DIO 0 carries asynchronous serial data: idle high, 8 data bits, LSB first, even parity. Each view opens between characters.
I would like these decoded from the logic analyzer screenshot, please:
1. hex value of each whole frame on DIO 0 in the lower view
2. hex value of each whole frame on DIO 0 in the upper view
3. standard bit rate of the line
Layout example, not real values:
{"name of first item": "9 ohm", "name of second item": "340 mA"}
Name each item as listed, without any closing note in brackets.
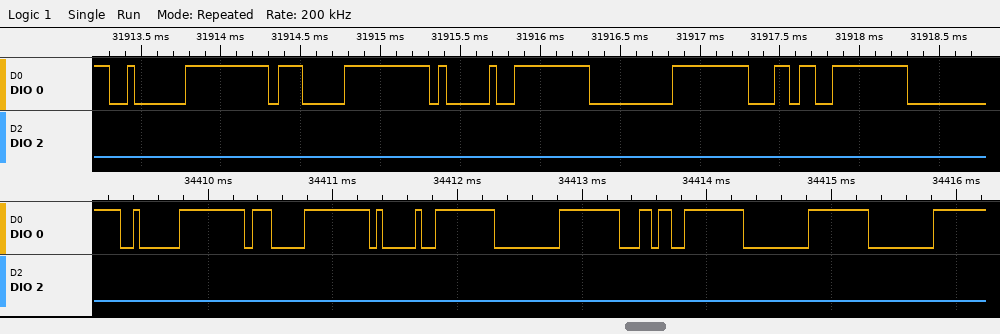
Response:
{"hex value of each whole frame on DIO 0 in the lower view": "02, 07, 41, 00, 6C, 00, 00", "hex value of each whole frame on DIO 0 in the upper view": "02, 07, 41, 00, 6C", "standard bit rate of the line": "19200 baud"}
